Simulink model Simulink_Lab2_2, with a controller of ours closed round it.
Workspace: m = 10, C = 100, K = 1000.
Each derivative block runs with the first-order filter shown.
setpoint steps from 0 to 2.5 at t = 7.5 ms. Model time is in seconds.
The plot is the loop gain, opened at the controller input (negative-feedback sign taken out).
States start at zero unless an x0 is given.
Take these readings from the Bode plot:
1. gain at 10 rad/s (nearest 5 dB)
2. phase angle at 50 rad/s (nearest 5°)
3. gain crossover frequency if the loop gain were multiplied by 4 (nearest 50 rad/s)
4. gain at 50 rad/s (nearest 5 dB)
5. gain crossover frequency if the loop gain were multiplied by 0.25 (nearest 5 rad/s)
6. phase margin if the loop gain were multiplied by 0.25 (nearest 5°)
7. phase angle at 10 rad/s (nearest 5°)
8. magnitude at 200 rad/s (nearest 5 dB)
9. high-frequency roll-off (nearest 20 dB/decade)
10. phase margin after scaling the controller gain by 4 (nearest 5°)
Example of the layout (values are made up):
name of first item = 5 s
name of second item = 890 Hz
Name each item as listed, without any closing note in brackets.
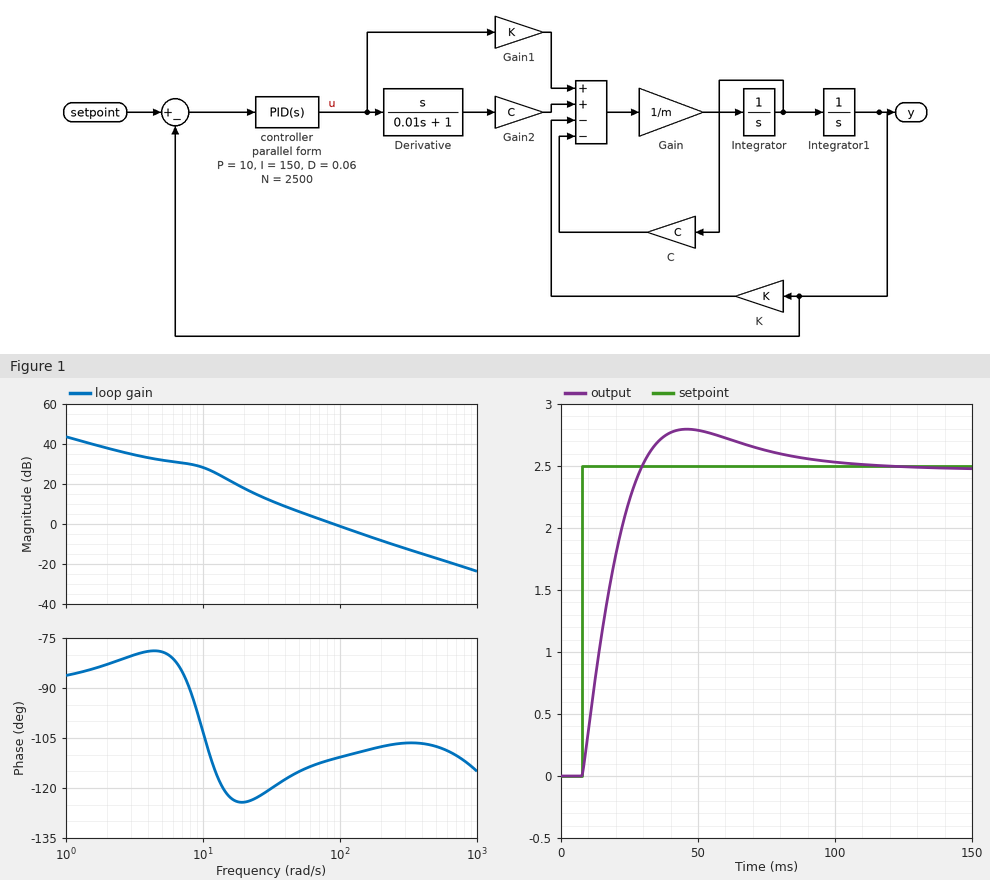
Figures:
gain at 10 rad/s = 30 dB
phase angle at 50 rad/s = -115°
gain crossover frequency if the loop gain were multiplied by 4 = 300 rad/s
gain at 50 rad/s = 5 dB
gain crossover frequency if the loop gain were multiplied by 0.25 = 30 rad/s
phase margin if the loop gain were multiplied by 0.25 = 60°
phase angle at 10 rad/s = -105°
magnitude at 200 rad/s = -10 dB
high-frequency roll-off = -20 dB/decade
phase margin after scaling the controller gain by 4 = 75°
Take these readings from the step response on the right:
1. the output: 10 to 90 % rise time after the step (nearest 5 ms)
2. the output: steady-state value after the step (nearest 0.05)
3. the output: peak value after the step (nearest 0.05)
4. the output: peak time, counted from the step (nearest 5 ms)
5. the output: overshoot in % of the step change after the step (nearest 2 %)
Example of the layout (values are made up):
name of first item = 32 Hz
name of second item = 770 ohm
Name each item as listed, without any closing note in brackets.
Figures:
the output: 10 to 90 % rise time after the step = 15 ms
the output: steady-state value after the step = 2.50
the output: peak value after the step = 2.80
the output: peak time, counted from the step = 40 ms
the output: overshoot in % of the step change after the step = 12 %
